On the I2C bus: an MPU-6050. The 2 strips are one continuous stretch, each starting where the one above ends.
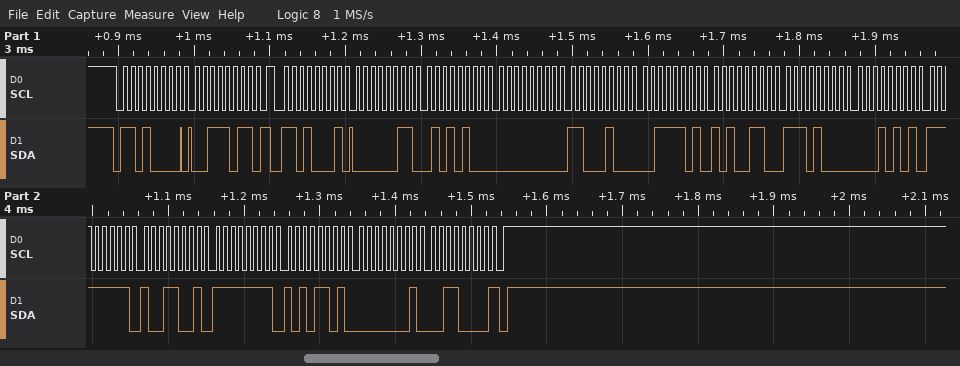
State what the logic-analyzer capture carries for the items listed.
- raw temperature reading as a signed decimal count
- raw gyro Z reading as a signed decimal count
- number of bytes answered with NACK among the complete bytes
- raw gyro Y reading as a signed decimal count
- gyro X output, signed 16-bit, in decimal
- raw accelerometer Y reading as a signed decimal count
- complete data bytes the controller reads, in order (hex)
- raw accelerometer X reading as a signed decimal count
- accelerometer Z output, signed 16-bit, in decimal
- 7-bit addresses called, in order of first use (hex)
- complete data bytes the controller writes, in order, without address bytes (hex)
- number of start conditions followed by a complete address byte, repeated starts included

-6123
304
1
-83
-103
196
03 54 00 C4 3D A6 E8 15 FF 99 FF AD 01 30
852
15782
0x68
3B
2
